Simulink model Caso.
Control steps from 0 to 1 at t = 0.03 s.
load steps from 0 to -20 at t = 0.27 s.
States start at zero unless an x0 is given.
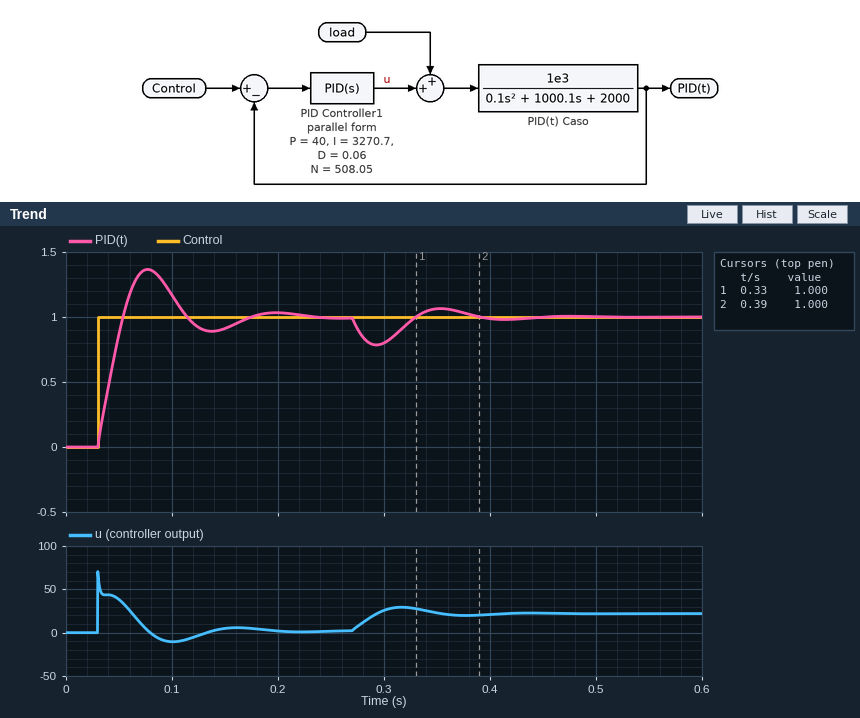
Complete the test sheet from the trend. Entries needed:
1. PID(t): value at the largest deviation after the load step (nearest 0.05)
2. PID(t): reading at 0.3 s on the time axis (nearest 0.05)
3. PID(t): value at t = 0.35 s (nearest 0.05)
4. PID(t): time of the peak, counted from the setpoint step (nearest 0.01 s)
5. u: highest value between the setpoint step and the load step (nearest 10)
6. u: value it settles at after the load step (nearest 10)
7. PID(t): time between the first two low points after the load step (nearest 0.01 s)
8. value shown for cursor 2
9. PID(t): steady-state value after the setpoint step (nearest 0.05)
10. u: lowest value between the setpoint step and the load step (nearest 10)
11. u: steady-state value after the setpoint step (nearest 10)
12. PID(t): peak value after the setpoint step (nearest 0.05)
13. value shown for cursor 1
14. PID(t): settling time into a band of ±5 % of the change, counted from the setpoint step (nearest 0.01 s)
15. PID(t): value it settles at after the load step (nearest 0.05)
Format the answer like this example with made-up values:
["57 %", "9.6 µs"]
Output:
["0.80", "0.80", "1.05", "0.05 s", "70", "20", "0.12 s", "1.000", "1.00", "-10", "0", "1.35", "1.000", "0.13 s", "1.00"]
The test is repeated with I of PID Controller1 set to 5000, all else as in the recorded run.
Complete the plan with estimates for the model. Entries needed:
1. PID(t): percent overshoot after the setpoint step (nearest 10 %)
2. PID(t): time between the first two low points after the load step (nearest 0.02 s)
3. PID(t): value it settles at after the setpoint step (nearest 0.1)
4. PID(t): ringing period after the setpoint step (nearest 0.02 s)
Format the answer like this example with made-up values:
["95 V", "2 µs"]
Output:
["40 %", "0.10 s", "1.0", "0.10 s"]
